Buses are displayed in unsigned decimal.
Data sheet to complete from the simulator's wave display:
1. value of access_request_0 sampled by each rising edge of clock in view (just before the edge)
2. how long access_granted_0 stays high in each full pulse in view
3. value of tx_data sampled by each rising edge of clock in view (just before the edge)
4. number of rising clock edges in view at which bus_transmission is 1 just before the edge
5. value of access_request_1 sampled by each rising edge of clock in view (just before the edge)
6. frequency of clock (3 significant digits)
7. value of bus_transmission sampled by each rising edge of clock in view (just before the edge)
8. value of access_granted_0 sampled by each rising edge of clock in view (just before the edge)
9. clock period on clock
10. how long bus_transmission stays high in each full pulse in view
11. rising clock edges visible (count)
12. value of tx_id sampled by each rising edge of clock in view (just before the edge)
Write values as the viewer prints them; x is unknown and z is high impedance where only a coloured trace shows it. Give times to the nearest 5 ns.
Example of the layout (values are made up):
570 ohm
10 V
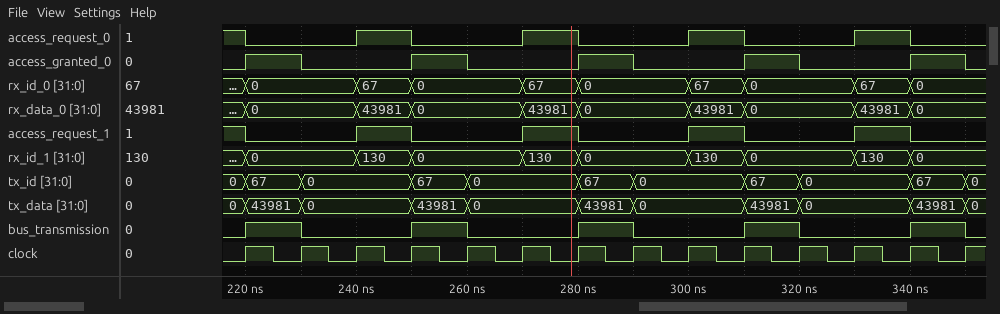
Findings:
1 0 0 1 0 0 1 0 0 1 0 0 1 0
10 ns, 10 ns, 10 ns, 10 ns, 10 ns
0, 43981, 0, 0, 43981, 0, 0, 43981, 0, 0, 43981, 0, 0, 43981
5
1 0 0 1 0 0 1 0 0 1 0 0 1 0
100 MHz
0 1 0 0 1 0 0 1 0 0 1 0 0 1
0 1 0 0 1 0 0 1 0 0 1 0 0 1
10 ns
10 ns, 10 ns, 10 ns, 10 ns, 10 ns
14
0, 67, 0, 0, 67, 0, 0, 67, 0, 0, 67, 0, 0, 67
